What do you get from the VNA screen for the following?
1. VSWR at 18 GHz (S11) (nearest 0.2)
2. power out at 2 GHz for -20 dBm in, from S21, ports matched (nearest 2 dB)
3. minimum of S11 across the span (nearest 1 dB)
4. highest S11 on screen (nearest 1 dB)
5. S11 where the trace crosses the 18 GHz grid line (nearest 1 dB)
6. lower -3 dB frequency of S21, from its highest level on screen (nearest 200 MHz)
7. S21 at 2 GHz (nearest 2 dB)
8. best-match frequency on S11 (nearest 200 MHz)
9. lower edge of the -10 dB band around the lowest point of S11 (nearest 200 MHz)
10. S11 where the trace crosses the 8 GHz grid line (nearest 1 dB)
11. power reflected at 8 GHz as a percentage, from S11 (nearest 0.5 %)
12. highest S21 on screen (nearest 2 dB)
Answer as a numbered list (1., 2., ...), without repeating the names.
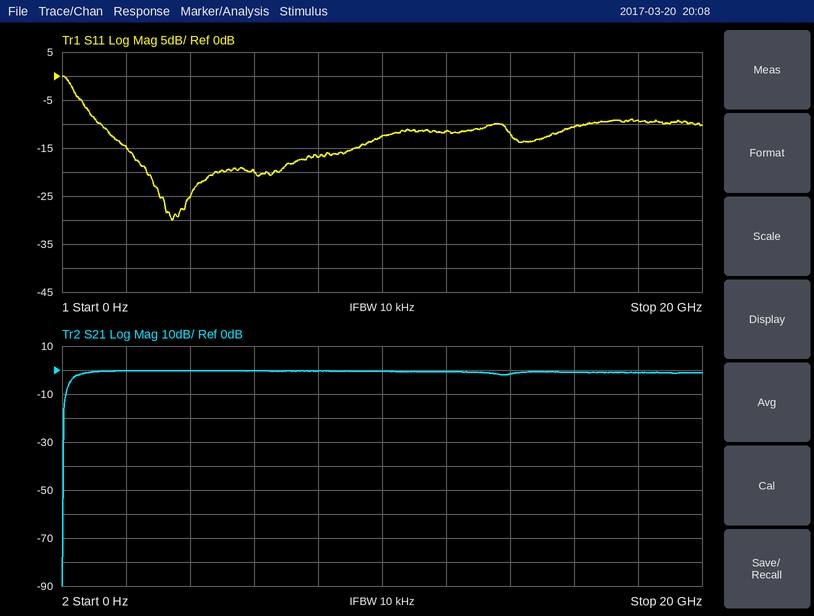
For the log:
1. 2.0
2. -20 dBm
3. -30 dB
4. 0 dB
5. -9 dB
6. 400 MHz
7. 0 dB
8. 3.4 GHz
9. 1.2 GHz
10. -17 dB
11. 2.0 %
12. 0 dB
